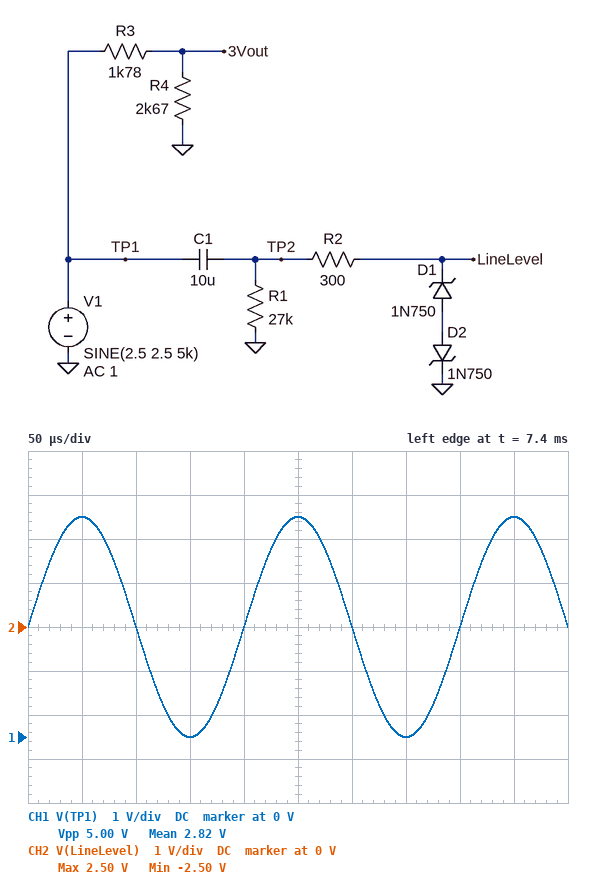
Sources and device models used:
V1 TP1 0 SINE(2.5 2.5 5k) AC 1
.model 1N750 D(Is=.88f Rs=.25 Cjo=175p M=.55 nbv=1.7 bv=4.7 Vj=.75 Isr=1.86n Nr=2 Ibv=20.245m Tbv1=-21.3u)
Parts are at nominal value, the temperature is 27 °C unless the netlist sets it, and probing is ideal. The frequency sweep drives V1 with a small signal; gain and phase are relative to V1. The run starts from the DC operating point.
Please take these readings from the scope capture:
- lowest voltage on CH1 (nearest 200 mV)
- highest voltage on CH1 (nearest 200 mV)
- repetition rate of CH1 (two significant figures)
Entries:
0 V
5.0 V
5.0 kHz
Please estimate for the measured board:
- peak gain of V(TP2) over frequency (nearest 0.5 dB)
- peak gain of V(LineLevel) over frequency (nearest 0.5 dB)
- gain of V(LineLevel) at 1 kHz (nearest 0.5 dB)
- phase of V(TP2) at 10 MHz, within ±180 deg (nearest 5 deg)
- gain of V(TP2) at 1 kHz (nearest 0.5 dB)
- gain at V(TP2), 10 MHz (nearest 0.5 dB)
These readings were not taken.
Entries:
0 dB
0 dB
0 dB
0 deg
0 dB
0 dB
